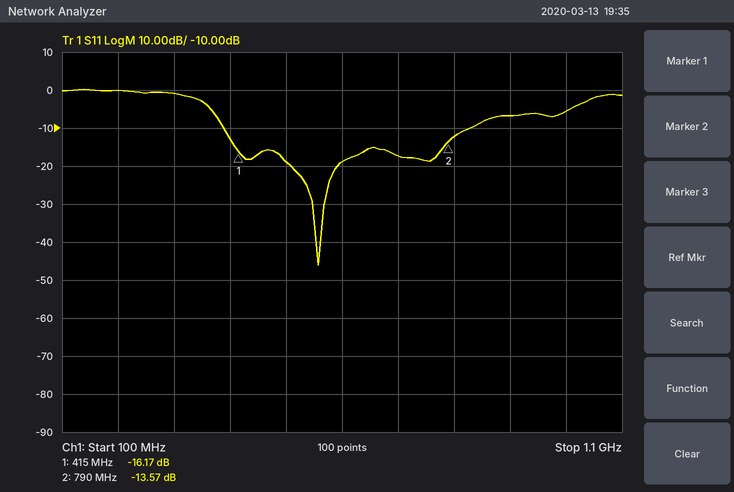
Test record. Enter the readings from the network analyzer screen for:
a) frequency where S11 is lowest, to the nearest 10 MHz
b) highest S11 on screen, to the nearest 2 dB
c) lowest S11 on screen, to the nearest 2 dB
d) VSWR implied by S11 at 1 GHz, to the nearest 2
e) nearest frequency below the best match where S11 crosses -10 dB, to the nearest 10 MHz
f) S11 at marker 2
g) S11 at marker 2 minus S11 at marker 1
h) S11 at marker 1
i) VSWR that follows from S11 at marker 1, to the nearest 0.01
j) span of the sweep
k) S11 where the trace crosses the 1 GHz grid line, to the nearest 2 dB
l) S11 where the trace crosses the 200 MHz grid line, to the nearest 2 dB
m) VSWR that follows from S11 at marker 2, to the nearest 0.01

560 MHz
0 dB
-46 dB
4
390 MHz
-13.57 dB
2.60 dB
-16.17 dB
1.37
1 GHz
-6 dB
0 dB
1.53
